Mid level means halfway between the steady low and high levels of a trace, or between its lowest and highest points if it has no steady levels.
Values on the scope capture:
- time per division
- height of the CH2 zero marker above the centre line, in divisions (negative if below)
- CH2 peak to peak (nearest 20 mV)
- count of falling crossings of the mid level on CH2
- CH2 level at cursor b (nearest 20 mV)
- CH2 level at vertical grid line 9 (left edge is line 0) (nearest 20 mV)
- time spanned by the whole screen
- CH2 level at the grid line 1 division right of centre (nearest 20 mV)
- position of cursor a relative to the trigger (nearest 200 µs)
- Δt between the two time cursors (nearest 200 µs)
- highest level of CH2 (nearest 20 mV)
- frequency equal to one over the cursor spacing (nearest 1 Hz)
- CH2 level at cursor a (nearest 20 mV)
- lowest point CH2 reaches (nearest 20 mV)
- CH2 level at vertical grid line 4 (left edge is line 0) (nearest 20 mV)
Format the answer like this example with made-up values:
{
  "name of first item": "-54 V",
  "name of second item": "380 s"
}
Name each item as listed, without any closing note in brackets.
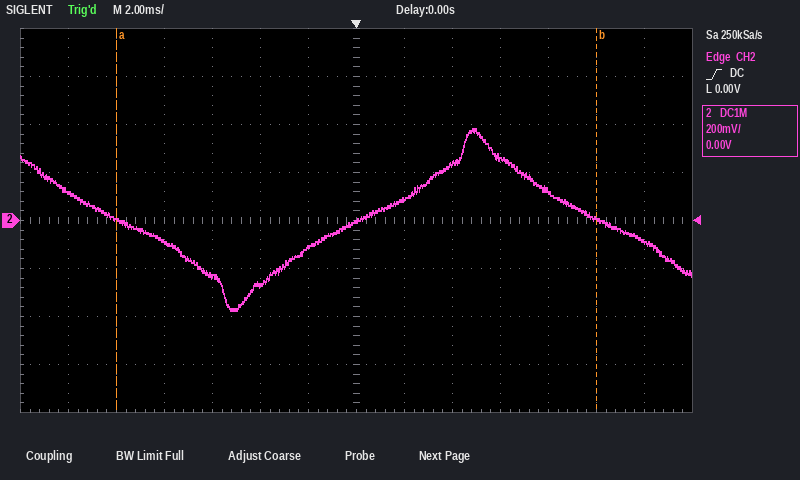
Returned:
{
  "time per division": "2 ms",
  "height of the CH2 zero marker above the centre line, in divisions": "0.0 div",
  "CH2 peak to peak": "760 mV",
  "count of falling crossings of the mid level on CH2": "2",
  "CH2 level at cursor b": "0 mV",
  "CH2 level at vertical grid line 9 (left edge is line 0)": "240 mV",
  "time spanned by the whole screen": "28 ms",
  "CH2 level at the grid line 1 division right of centre": "80 mV",
  "position of cursor a relative to the trigger": "-10.0 ms",
  "Δt between the two time cursors": "20.0 ms",
  "highest level of CH2": "380 mV",
  "frequency equal to one over the cursor spacing": "50 Hz",
  "CH2 level at cursor a": "0 mV",
  "lowest point CH2 reaches": "-380 mV",
  "CH2 level at vertical grid line 4 (left edge is line 0)": "-220 mV"
}
